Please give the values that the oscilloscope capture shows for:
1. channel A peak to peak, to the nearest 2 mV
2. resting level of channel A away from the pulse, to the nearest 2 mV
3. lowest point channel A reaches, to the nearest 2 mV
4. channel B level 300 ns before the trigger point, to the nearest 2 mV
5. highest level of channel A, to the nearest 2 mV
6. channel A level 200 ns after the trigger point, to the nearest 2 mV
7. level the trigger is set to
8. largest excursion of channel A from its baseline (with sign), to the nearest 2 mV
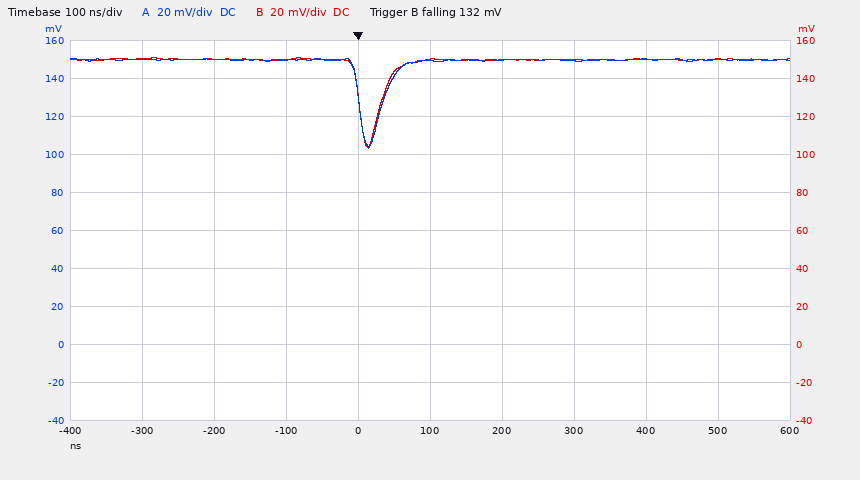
46 mV
150 mV
104 mV
150 mV
150 mV
150 mV
132 mV
-46 mV
